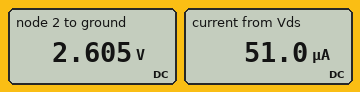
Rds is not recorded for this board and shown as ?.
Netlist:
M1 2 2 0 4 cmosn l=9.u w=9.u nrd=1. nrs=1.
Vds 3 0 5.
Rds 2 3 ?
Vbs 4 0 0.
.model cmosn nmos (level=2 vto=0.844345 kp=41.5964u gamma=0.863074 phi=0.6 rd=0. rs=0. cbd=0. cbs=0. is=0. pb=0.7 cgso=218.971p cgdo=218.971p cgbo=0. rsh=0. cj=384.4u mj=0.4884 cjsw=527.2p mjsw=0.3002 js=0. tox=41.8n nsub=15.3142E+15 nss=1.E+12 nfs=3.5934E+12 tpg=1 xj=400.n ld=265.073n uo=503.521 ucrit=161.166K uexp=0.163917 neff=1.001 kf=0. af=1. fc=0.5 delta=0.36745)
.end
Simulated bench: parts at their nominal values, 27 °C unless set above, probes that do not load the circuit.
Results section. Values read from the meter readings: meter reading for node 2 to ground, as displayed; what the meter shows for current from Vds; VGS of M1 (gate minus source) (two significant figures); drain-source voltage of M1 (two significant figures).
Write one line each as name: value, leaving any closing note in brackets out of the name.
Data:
meter reading for node 2 to ground, as displayed: 2.605 V
what the meter shows for current from Vds: 51.0 µA
VGS of M1 (gate minus source): 2.6 V
drain-source voltage of M1: 2.6 V
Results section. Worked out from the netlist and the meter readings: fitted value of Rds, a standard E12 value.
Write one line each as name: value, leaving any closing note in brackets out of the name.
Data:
fitted value of Rds, a standard E12 value: 47 kΩ
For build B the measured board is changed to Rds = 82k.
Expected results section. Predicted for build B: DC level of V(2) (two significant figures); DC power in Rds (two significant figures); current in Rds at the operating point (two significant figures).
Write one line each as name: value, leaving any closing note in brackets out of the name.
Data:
DC level of V(2): 2.3 V
DC power in Rds: 91 µW
current in Rds at the operating point: 33 µA
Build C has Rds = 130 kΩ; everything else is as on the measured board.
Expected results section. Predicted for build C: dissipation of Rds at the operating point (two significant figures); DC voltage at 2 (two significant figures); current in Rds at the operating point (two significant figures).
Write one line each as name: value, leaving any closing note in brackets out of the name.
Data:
dissipation of Rds at the operating point: 68 µW
DC voltage at 2: 2.0 V
current in Rds at the operating point: 23 µA
